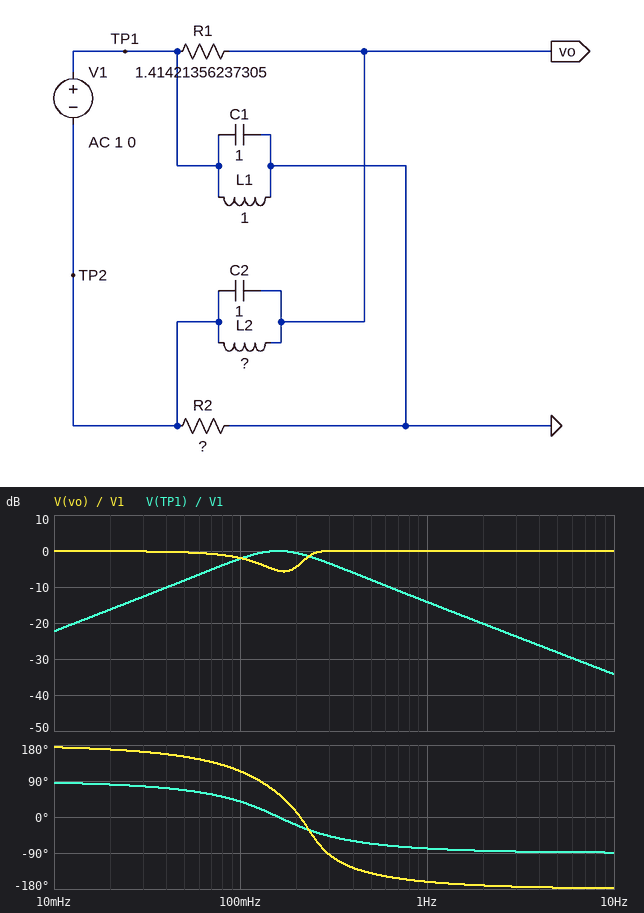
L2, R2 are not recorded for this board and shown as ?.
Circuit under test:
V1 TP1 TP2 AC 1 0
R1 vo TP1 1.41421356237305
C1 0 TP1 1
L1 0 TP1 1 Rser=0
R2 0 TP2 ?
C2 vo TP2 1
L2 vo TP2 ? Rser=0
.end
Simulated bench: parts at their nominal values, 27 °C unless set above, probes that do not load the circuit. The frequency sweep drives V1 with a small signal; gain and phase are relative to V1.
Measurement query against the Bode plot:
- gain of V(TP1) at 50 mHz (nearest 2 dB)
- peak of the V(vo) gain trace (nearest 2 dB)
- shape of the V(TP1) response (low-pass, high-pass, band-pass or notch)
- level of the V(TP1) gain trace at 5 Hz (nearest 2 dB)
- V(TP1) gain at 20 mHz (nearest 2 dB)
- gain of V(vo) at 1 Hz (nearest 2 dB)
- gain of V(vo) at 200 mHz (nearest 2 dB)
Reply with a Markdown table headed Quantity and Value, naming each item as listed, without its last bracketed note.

| Quantity | Value |
|---|---|
| gain of V(TP1) at 50 mHz | -8 dB |
| peak of the V(vo) gain trace | 0 dB |
| shape of the V(TP1) response | band-pass |
| level of the V(TP1) gain trace at 5 Hz | -28 dB |
| V(TP1) gain at 20 mHz | -16 dB |
| gain of V(vo) at 1 Hz | 0 dB |
| gain of V(vo) at 200 mHz | -4 dB |
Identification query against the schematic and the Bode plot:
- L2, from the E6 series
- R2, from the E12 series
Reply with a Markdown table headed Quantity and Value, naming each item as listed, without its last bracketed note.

| Quantity | Value |
|---|---|
| L2, from the E6 series | 470 mH |
| R2, from the E12 series | 0.82 Ω |
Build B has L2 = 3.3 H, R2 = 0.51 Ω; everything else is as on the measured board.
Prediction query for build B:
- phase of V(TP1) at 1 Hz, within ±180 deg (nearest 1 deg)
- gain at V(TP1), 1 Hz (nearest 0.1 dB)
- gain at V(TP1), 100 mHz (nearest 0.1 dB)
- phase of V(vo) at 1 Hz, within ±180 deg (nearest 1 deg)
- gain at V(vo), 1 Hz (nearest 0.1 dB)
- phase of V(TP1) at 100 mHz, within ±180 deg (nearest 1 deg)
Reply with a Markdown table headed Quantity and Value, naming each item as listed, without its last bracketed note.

| Quantity | Value |
|---|---|
| phase of V(TP1) at 1 Hz, within ±180 deg | -72 deg |
| gain at V(TP1), 1 Hz | -10.3 dB |
| gain at V(TP1), 100 mHz | -0.9 dB |
| phase of V(vo) at 1 Hz, within ±180 deg | -156 deg |
| gain at V(vo), 1 Hz | -0.2 dB |
| phase of V(TP1) at 100 mHz, within ±180 deg | 26 deg |
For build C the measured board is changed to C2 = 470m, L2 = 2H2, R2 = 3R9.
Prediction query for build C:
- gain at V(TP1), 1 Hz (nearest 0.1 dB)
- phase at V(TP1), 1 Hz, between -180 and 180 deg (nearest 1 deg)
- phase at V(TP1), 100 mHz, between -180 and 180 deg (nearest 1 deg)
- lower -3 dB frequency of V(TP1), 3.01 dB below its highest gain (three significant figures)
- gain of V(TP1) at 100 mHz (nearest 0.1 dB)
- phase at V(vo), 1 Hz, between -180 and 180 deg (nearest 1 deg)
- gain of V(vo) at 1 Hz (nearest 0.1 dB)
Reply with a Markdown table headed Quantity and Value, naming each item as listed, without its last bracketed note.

| Quantity | Value |
|---|---|
| gain at V(TP1), 1 Hz | -27.6 dB |
| phase at V(TP1), 1 Hz, between -180 and 180 deg | -88 deg |
| phase at V(TP1), 100 mHz, between -180 and 180 deg | 75 deg |
| lower -3 dB frequency of V(TP1), 3.01 dB below its highest gain | 140 mHz |
| gain of V(TP1) at 100 mHz | -11.8 dB |
| phase at V(vo), 1 Hz, between -180 and 180 deg | -164 deg |
| gain of V(vo) at 1 Hz | -0.2 dB |
